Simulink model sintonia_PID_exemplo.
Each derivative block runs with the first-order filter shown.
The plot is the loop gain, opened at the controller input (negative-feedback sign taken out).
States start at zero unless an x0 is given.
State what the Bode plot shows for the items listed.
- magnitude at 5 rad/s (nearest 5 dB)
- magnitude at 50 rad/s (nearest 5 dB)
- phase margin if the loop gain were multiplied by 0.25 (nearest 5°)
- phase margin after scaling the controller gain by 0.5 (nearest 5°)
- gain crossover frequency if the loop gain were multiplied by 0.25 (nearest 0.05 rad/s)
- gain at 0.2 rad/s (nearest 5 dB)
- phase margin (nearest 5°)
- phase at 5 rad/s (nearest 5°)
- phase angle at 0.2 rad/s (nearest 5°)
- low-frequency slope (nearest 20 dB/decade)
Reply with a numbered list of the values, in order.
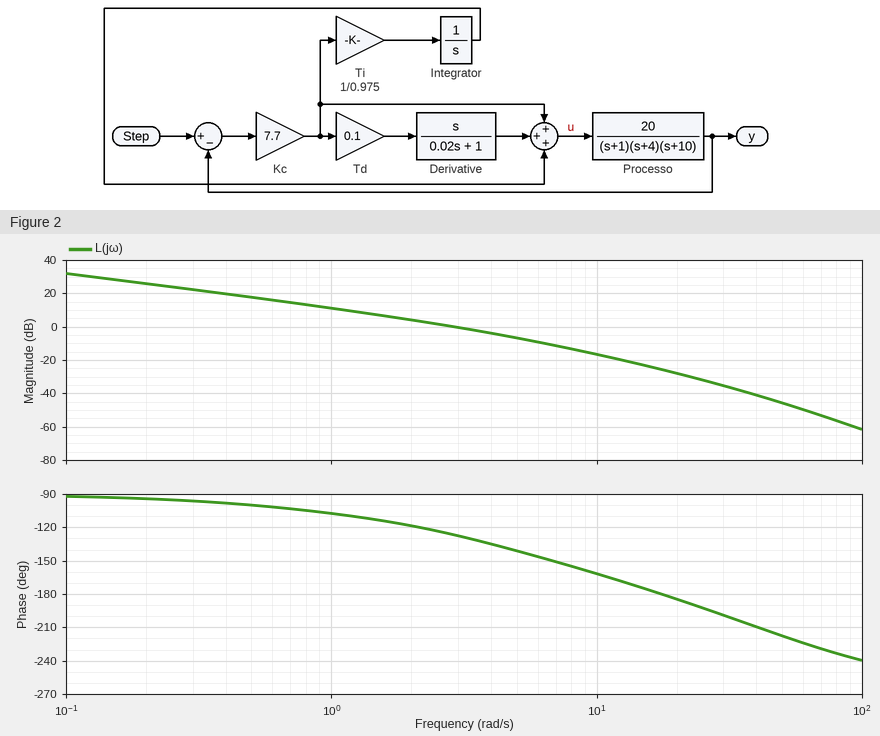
1. -5 dB
2. -45 dB
3. 75°
4. 65°
5. 0.90 rad/s
6. 25 dB
7. 55°
8. -140°
9. -95°
10. -20 dB/decade
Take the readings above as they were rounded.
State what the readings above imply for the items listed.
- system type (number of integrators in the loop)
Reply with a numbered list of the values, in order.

1. 1
